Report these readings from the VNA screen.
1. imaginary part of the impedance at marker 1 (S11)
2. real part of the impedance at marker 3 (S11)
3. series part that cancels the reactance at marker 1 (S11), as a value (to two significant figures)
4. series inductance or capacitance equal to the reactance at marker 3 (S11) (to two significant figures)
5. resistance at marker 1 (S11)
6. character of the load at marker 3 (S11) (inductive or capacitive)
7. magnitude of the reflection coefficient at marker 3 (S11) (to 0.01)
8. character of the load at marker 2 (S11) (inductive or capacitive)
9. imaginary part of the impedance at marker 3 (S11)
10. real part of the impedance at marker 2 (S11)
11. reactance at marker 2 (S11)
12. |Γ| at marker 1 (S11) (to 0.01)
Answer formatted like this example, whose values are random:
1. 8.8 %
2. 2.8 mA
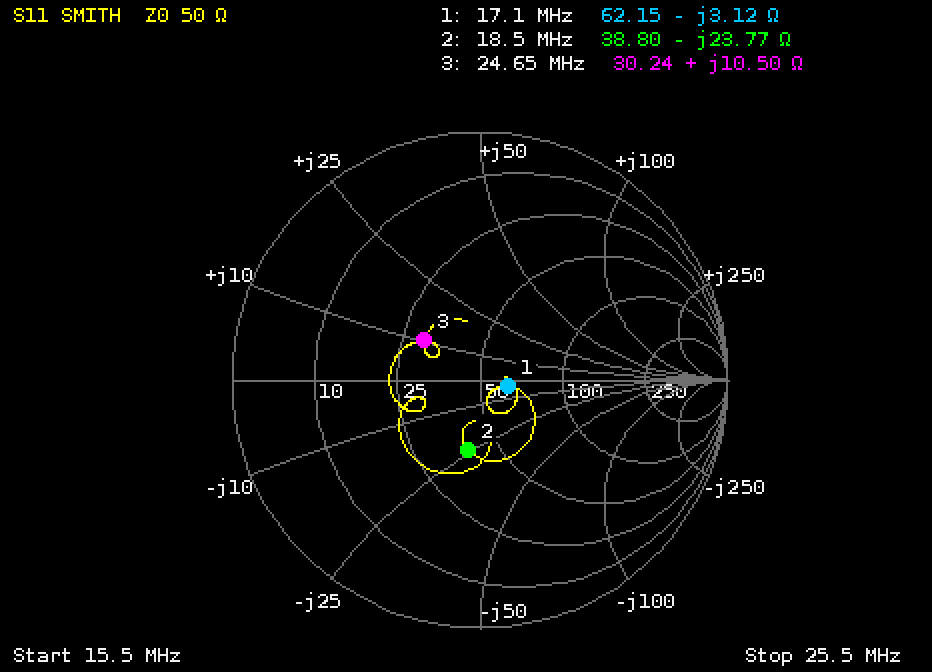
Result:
1. -3.12 Ω
2. 30.24 Ω
3. 29 nH
4. 68 nH
5. 62.15 Ω
6. inductive
7. 0.28
8. capacitive
9. +10.50 Ω
10. 38.80 Ω
11. -23.77 Ω
12. 0.11
